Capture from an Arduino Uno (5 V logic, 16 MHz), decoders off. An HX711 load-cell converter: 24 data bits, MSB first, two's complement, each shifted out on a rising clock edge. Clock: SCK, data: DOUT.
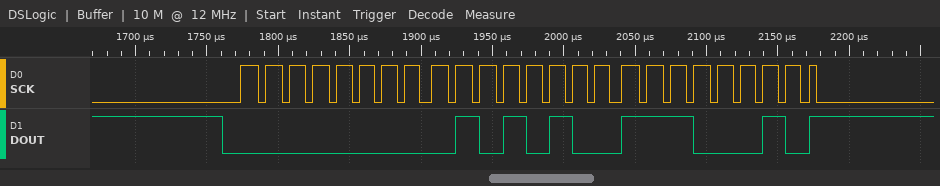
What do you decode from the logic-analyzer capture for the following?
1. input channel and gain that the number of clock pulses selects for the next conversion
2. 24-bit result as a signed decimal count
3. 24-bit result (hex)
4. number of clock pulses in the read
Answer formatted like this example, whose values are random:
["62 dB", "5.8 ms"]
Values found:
["channel A, gain 128", "21730", "0x0054E2", "25"]
